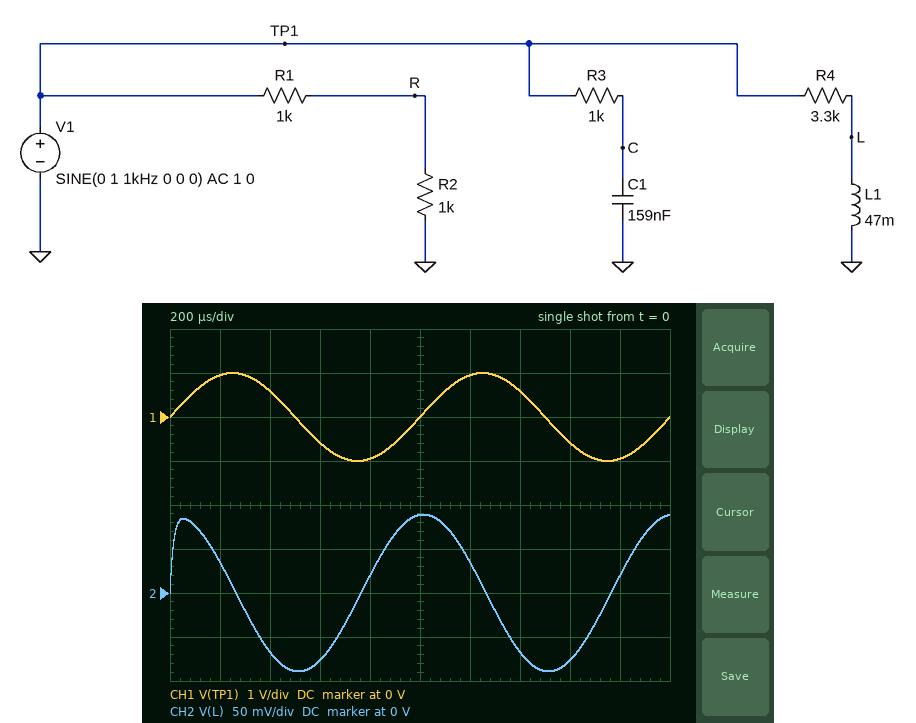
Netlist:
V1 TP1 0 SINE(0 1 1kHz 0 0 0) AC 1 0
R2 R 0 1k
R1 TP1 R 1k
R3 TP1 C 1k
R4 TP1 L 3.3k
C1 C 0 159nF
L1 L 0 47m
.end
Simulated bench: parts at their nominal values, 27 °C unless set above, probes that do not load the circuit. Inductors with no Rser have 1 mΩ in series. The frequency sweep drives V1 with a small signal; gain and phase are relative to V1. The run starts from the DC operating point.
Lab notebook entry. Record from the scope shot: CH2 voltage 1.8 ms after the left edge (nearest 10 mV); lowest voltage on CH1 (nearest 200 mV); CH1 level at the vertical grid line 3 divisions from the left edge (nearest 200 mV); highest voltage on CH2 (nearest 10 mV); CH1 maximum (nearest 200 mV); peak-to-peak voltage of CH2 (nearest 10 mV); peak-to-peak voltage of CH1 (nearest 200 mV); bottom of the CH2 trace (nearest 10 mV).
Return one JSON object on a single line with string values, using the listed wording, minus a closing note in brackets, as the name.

{"CH2 voltage 1.8 ms after the left edge": "20 mV", "lowest voltage on CH1": "-1.0 V", "CH1 level at the vertical grid line 3 divisions from the left edge": "-600 mV", "highest voltage on CH2": "90 mV", "CH1 maximum": "1.0 V", "peak-to-peak voltage of CH2": "180 mV", "peak-to-peak voltage of CH1": "2.0 V", "bottom of the CH2 trace": "-90 mV"}
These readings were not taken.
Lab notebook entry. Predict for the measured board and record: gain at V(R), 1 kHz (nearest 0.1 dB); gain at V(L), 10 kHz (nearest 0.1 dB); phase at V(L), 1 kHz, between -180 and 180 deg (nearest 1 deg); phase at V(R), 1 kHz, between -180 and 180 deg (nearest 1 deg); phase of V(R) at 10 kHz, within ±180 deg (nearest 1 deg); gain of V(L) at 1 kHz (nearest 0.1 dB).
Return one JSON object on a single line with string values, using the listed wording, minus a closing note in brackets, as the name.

{"gain at V(R), 1 kHz": "-6.0 dB", "gain at V(L), 10 kHz": "-3.5 dB", "phase at V(L), 1 kHz, between -180 and 180 deg": "85 deg", "phase at V(R), 1 kHz, between -180 and 180 deg": "0 deg", "phase of V(R) at 10 kHz, within ±180 deg": "0 deg", "gain of V(L) at 1 kHz": "-21.0 dB"}
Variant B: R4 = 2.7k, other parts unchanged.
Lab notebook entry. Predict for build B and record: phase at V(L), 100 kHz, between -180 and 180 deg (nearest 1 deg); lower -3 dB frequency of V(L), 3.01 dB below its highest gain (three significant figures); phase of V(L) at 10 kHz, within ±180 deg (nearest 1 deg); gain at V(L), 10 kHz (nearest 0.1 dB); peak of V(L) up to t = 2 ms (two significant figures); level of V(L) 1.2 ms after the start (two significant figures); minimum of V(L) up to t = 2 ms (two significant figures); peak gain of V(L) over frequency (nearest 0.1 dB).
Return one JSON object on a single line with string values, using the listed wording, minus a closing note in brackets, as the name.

{"phase at V(L), 100 kHz, between -180 and 180 deg": "5 deg", "lower -3 dB frequency of V(L), 3.01 dB below its highest gain": "9.14 kHz", "phase of V(L) at 10 kHz, within ±180 deg": "42 deg", "gain at V(L), 10 kHz": "-2.6 dB", "peak of V(L) up to t = 2 ms": "110 mV", "level of V(L) 1.2 ms after the start": "45 mV", "minimum of V(L) up to t = 2 ms": "-110 mV", "peak gain of V(L) over frequency": "0 dB"}
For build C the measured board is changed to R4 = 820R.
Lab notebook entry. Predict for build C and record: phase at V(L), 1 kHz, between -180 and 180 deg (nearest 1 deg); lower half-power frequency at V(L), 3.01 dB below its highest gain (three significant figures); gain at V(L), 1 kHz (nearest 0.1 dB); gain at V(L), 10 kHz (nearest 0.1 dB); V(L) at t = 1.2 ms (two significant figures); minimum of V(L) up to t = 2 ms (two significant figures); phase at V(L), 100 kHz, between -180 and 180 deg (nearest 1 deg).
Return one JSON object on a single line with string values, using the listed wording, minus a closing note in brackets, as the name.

{"phase at V(L), 1 kHz, between -180 and 180 deg": "70 deg", "lower half-power frequency at V(L), 3.01 dB below its highest gain": "2.78 kHz", "gain at V(L), 1 kHz": "-9.4 dB", "gain at V(L), 10 kHz": "-0.3 dB", "V(L) at t = 1.2 ms": "210 mV", "minimum of V(L) up to t = 2 ms": "-340 mV", "phase at V(L), 100 kHz, between -180 and 180 deg": "2 deg"}
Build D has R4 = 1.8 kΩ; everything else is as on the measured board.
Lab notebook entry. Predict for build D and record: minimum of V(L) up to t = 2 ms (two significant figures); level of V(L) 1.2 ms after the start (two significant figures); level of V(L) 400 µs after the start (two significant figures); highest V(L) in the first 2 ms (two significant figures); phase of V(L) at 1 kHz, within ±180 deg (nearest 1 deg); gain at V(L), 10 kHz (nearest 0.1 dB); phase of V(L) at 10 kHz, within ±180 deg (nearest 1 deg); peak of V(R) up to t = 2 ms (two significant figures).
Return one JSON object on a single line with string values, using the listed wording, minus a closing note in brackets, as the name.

{"minimum of V(L) up to t = 2 ms": "-160 mV", "level of V(L) 1.2 ms after the start": "74 mV", "level of V(L) 400 µs after the start": "-110 mV", "highest V(L) in the first 2 ms": "160 mV", "phase of V(L) at 1 kHz, within ±180 deg": "81 deg", "gain at V(L), 10 kHz": "-1.4 dB", "phase of V(L) at 10 kHz, within ±180 deg": "31 deg", "peak of V(R) up to t = 2 ms": "500 mV"}
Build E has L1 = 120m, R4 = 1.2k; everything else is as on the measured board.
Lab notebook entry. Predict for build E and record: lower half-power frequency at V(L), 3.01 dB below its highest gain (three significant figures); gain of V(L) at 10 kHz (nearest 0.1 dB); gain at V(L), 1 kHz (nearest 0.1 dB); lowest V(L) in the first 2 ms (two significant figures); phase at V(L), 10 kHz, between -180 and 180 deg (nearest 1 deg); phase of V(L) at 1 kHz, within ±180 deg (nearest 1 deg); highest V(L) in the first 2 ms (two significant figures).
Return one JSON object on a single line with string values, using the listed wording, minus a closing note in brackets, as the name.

{"lower half-power frequency at V(L), 3.01 dB below its highest gain": "1.59 kHz", "gain of V(L) at 10 kHz": "-0.1 dB", "gain at V(L), 1 kHz": "-5.5 dB", "lowest V(L) in the first 2 ms": "-530 mV", "phase at V(L), 10 kHz, between -180 and 180 deg": "9 deg", "phase of V(L) at 1 kHz, within ±180 deg": "58 deg", "highest V(L) in the first 2 ms": "530 mV"}
